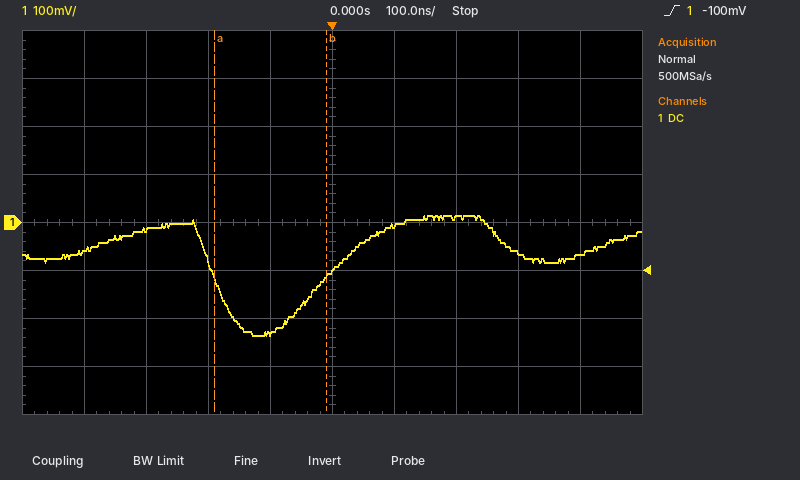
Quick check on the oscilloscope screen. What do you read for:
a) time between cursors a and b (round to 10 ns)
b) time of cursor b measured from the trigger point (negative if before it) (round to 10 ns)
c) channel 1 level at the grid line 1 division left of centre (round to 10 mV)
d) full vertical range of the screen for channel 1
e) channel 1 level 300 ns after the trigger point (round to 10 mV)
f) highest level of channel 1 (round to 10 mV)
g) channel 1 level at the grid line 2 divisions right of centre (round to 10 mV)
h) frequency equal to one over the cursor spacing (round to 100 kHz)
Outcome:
180 ns
-10 ns
-230 mV
800 mV
-60 mV
10 mV
10 mV
5.6 MHz
